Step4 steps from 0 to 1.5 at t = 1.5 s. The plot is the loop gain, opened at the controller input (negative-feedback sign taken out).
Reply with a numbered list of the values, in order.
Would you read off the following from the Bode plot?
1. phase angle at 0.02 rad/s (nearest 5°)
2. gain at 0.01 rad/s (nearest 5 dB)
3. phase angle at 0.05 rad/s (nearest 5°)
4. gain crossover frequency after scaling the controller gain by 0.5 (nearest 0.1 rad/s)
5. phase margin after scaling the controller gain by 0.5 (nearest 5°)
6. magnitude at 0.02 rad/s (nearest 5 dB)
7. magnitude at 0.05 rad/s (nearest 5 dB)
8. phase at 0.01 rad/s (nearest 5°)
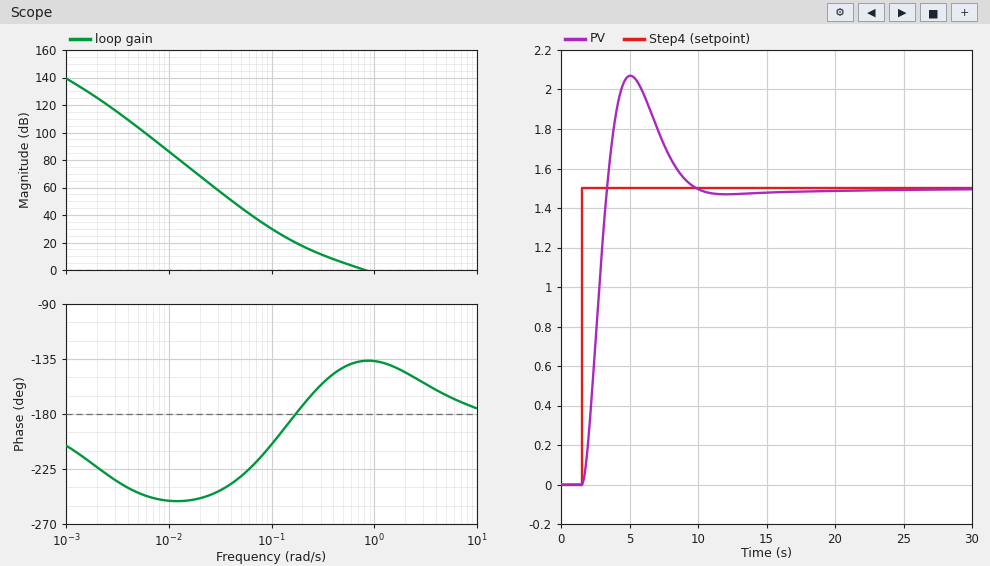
1. -250°
2. 85 dB
3. -230°
4. 0.5 rad/s
5. 35°
6. 70 dB
7. 45 dB
8. -250°
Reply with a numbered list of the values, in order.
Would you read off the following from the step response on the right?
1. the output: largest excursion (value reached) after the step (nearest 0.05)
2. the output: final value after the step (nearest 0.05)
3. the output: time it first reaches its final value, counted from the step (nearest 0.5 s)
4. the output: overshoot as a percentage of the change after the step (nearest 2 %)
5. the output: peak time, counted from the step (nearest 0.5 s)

1. 2.05
2. 1.50
3. 2.0 s
4. 38 %
5. 3.5 s
